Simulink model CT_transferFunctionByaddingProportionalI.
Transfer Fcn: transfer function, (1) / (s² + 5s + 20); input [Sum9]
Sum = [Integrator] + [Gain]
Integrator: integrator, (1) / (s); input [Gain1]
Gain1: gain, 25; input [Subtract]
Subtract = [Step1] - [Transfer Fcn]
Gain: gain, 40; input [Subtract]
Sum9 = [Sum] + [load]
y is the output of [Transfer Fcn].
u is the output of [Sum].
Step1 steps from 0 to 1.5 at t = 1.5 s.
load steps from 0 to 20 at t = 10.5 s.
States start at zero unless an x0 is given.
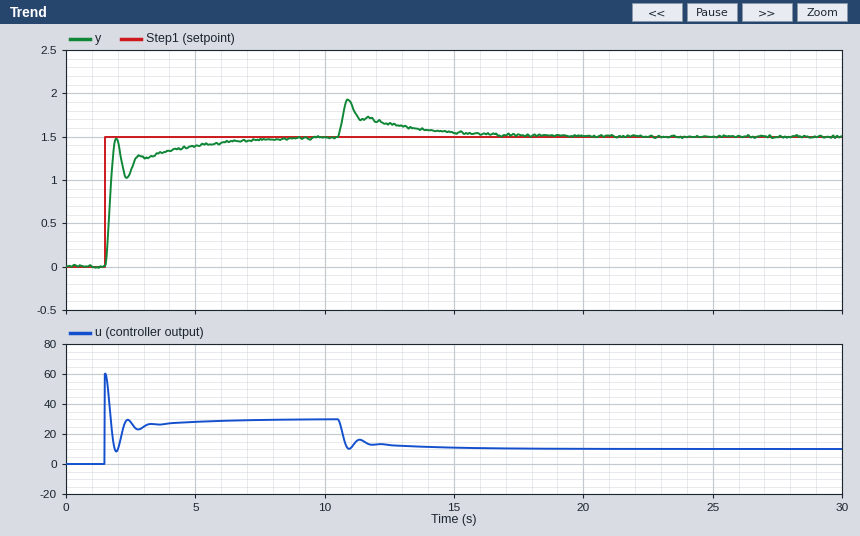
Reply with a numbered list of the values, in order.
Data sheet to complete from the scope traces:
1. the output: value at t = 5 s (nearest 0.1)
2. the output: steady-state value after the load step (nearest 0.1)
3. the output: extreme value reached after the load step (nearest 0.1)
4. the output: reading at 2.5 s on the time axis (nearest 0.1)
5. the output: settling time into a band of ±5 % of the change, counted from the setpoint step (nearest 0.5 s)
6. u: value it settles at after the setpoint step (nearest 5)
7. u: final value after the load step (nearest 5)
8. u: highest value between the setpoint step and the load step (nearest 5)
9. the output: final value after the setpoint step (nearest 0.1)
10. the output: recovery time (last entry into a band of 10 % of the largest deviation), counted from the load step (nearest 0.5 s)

1. 1.4
2. 1.5
3. 1.9
4. 1.1
5. 4.5 s
6. 30
7. 10
8. 60
9. 1.5
10. 5.0 s
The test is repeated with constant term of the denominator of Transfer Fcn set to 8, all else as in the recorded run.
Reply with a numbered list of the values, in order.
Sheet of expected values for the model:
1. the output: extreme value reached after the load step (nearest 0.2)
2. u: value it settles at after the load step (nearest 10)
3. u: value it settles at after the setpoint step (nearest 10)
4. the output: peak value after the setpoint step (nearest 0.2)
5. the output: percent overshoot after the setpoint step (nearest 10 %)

1. 2.0
2. -10
3. 10
4. 1.8
5. 20 %
